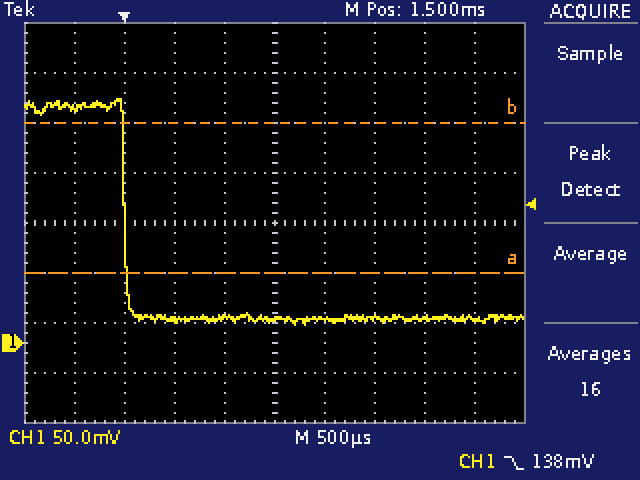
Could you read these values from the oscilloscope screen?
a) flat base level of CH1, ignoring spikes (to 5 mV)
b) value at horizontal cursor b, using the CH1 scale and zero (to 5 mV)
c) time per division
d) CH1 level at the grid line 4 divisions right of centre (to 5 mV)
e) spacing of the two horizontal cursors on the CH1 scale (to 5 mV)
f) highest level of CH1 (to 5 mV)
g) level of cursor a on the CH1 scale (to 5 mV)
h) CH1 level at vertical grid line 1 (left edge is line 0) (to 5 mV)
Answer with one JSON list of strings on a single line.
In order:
["25 mV", "220 mV", "500 µs", "25 mV", "150 mV", "245 mV", "70 mV", "235 mV"]
